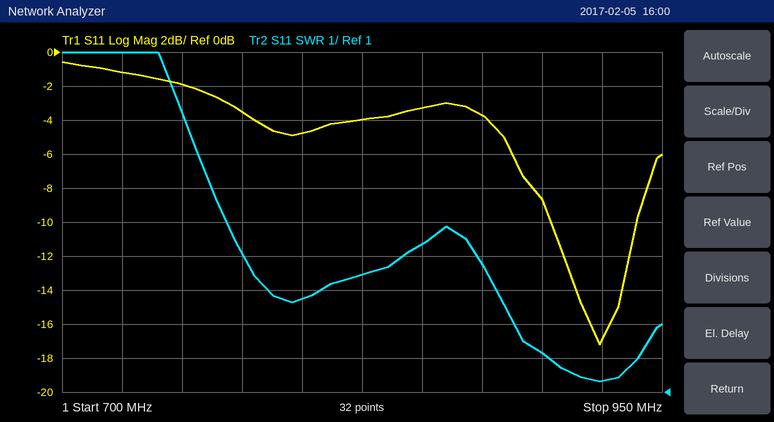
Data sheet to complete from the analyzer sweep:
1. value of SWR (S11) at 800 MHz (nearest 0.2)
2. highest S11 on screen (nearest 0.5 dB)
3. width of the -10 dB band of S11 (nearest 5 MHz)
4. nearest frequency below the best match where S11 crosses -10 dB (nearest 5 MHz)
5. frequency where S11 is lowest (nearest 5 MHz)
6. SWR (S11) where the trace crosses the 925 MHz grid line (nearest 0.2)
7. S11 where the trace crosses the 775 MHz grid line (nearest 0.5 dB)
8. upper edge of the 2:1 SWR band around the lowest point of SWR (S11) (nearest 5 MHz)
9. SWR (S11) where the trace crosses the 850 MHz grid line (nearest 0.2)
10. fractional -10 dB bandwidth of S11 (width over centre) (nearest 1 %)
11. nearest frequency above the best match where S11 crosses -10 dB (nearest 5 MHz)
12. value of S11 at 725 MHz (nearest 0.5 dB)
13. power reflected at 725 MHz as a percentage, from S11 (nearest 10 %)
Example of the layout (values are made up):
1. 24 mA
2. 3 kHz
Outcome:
1. 3.8
2. -0.5 dB
3. 35 MHz
4. 905 MHz
5. 925 MHz
6. 1.4
7. -3.5 dB
8. 940 MHz
9. 5.4
10. 4 %
11. 940 MHz
12. -1.0 dB
13. 80 %
